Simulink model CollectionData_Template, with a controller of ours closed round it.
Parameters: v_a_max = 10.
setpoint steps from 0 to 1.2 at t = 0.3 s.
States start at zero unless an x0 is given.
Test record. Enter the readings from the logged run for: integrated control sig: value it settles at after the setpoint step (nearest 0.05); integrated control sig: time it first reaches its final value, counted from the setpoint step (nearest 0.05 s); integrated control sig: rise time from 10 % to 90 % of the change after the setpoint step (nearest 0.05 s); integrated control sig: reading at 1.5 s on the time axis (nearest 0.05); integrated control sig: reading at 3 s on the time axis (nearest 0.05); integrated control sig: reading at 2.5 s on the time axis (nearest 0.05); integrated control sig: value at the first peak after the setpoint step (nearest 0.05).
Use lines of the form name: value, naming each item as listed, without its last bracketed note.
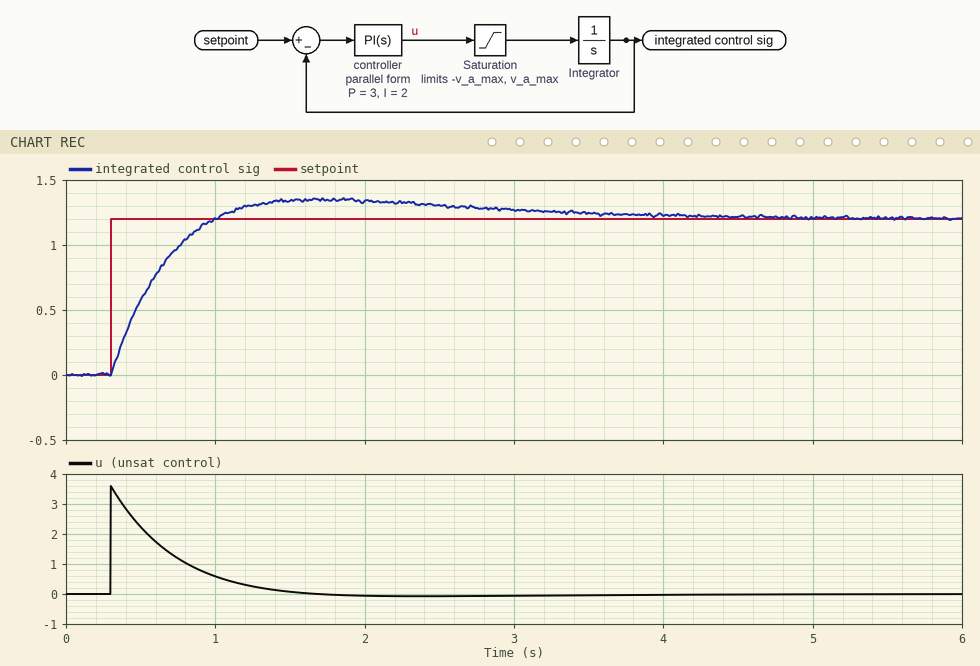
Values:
integrated control sig: value it settles at after the setpoint step: 1.20
integrated control sig: time it first reaches its final value, counted from the setpoint step: 0.70 s
integrated control sig: rise time from 10 % to 90 % of the change after the setpoint step: 0.50 s
integrated control sig: reading at 1.5 s on the time axis: 1.35
integrated control sig: reading at 3 s on the time axis: 1.25
integrated control sig: reading at 2.5 s on the time axis: 1.30
integrated control sig: value at the first peak after the setpoint step: 1.35
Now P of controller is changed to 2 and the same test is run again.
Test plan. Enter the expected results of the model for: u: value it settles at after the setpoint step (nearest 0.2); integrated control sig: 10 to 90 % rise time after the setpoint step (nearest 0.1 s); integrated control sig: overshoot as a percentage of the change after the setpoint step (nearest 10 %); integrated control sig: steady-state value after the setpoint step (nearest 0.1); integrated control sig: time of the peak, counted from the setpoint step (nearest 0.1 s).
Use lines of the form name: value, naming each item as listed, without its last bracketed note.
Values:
u: value it settles at after the setpoint step: 0.0
integrated control sig: 10 to 90 % rise time after the setpoint step: 0.6 s
integrated control sig: overshoot as a percentage of the change after the setpoint step: 20 %
integrated control sig: steady-state value after the setpoint step: 1.2
integrated control sig: time of the peak, counted from the setpoint step: 1.6 s
